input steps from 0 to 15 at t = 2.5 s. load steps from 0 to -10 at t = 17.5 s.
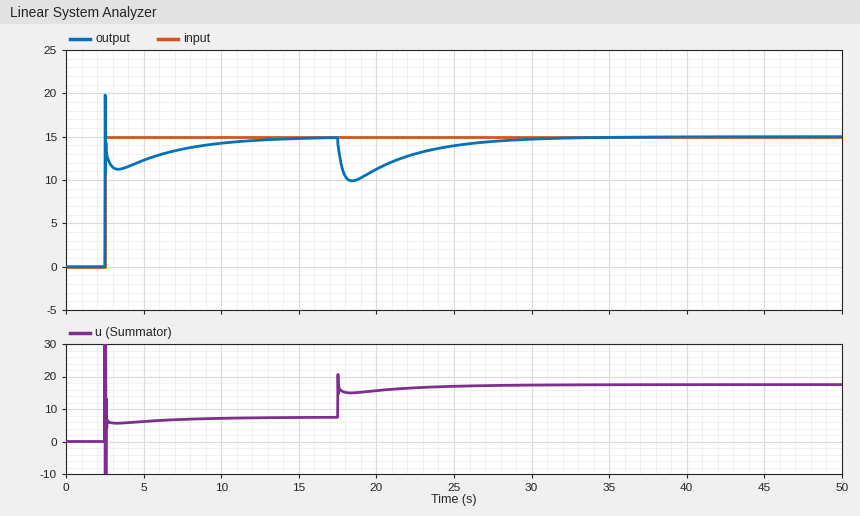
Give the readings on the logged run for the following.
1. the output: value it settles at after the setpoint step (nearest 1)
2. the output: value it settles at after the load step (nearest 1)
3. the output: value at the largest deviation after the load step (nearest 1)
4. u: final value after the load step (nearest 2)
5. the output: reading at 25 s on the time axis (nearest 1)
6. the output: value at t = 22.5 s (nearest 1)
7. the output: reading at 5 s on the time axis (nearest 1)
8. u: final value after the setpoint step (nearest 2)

15
15
10
18
14
13
12
8
